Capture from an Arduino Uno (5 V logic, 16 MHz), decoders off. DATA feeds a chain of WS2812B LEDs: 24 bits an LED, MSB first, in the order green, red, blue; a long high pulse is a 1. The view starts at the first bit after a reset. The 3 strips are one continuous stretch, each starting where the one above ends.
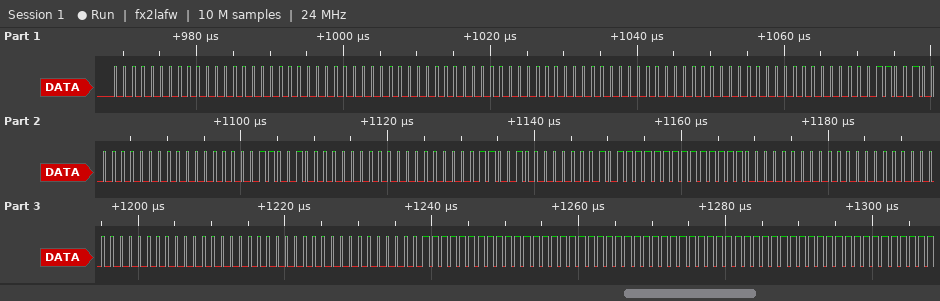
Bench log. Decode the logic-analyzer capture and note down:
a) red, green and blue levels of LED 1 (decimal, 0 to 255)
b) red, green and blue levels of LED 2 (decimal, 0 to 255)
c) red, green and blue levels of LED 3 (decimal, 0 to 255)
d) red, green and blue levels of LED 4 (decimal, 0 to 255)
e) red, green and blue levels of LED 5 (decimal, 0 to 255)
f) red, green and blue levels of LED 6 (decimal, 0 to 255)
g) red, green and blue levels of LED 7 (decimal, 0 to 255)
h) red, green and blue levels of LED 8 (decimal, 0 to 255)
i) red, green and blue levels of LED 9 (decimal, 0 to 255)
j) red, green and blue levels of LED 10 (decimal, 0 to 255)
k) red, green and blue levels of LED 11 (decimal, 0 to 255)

0, 0, 0
0, 0, 0
0, 0, 0
25, 0, 0
25, 0, 0
25, 0, 0
255, 191, 0
0, 0, 0
0, 0, 0
255, 255, 255
255, 255, 255
